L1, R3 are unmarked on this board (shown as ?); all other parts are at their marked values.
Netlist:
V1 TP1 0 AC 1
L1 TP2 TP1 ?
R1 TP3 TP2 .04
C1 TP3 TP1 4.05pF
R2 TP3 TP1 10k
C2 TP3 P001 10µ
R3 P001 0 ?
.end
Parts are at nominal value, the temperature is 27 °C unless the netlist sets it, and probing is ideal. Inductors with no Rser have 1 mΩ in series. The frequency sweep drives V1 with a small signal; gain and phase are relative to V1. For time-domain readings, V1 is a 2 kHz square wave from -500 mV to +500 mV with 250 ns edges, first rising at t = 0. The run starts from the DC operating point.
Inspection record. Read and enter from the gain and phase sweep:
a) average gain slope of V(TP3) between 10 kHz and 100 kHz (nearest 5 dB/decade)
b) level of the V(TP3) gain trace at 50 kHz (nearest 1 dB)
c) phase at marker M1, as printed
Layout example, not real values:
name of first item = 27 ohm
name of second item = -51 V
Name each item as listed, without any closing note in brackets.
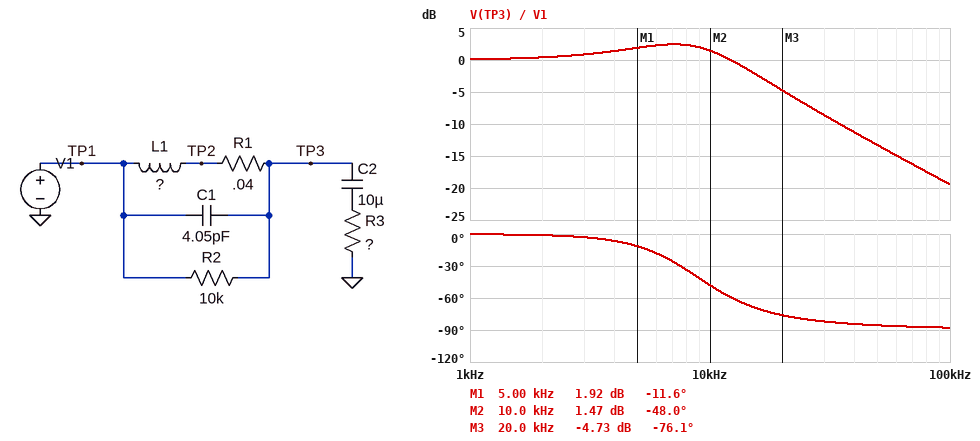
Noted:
average gain slope of V(TP3) between 10 kHz and 100 kHz = -20 dB/decade
level of the V(TP3) gain trace at 50 kHz = -13 dB
phase at marker M1, as printed = -11.6 deg
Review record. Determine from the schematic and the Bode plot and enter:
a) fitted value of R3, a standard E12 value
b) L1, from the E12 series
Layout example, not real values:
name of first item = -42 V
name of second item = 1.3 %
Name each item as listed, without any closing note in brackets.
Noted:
fitted value of R3, a standard E12 value = 2.2 Ω
L1, from the E12 series = 33 µH
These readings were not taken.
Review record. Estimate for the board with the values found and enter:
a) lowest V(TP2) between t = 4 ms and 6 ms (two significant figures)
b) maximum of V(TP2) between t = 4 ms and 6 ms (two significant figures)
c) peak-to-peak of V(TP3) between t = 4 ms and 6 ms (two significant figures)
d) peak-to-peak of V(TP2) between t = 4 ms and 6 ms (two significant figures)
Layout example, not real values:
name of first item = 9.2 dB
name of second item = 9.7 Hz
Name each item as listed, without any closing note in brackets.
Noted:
lowest V(TP2) between t = 4 ms and 6 ms = -740 mV
maximum of V(TP2) between t = 4 ms and 6 ms = 740 mV
peak-to-peak of V(TP3) between t = 4 ms and 6 ms = 1.5 V
peak-to-peak of V(TP2) between t = 4 ms and 6 ms = 1.5 V
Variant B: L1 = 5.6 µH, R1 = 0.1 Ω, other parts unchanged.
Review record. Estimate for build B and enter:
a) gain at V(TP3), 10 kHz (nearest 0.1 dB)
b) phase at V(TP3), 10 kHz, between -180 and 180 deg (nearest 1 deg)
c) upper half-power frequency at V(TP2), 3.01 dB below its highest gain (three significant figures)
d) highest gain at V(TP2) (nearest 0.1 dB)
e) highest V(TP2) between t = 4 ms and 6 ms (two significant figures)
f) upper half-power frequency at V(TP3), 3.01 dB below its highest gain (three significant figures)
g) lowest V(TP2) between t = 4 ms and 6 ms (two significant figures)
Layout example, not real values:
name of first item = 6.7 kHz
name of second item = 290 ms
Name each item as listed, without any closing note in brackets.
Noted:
gain at V(TP3), 10 kHz = 0.3 dB
phase at V(TP3), 10 kHz, between -180 and 180 deg = -8 deg
upper half-power frequency at V(TP2), 3.01 dB below its highest gain = 63.8 kHz
highest gain at V(TP2) = 0.6 dB
highest V(TP2) between t = 4 ms and 6 ms = 570 mV
upper half-power frequency at V(TP3), 3.01 dB below its highest gain = 62.5 kHz
lowest V(TP2) between t = 4 ms and 6 ms = -570 mV
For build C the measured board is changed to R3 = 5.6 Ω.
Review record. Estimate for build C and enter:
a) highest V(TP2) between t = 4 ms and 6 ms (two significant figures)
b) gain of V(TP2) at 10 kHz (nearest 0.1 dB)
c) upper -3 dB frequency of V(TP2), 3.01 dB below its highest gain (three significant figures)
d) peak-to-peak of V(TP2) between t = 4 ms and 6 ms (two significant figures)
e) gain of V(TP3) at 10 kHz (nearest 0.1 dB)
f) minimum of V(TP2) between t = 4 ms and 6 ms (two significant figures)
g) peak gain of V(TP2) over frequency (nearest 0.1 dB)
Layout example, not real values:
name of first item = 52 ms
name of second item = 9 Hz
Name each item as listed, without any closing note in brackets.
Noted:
highest V(TP2) between t = 4 ms and 6 ms = 570 mV
gain of V(TP2) at 10 kHz = 0.3 dB
upper -3 dB frequency of V(TP2), 3.01 dB below its highest gain = 26.5 kHz
peak-to-peak of V(TP2) between t = 4 ms and 6 ms = 1.1 V
gain of V(TP3) at 10 kHz = 0.2 dB
minimum of V(TP2) between t = 4 ms and 6 ms = -570 mV
peak gain of V(TP2) over frequency = 0.6 dB
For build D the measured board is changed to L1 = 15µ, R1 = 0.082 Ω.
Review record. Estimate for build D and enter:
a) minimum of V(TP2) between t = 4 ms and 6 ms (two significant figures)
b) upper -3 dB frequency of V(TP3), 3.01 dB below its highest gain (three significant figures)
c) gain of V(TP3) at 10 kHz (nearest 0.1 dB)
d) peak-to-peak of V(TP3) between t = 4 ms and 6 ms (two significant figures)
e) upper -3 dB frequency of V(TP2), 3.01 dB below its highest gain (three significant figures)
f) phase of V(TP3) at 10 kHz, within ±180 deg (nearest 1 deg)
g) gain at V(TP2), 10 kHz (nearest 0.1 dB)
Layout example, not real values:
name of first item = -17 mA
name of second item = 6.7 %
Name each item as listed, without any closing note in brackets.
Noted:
minimum of V(TP2) between t = 4 ms and 6 ms = -650 mV
upper -3 dB frequency of V(TP3), 3.01 dB below its highest gain = 24.6 kHz
gain of V(TP3) at 10 kHz = 1.2 dB
peak-to-peak of V(TP3) between t = 4 ms and 6 ms = 1.3 V
upper -3 dB frequency of V(TP2), 3.01 dB below its highest gain = 25.0 kHz
phase of V(TP3) at 10 kHz, within ±180 deg = -20 deg
gain at V(TP2), 10 kHz = 1.4 dB
